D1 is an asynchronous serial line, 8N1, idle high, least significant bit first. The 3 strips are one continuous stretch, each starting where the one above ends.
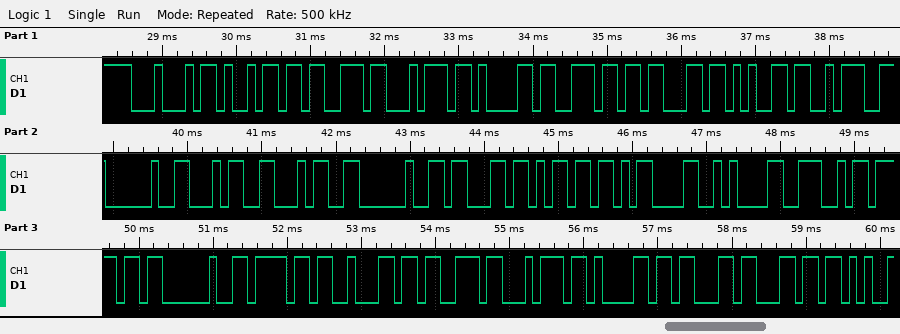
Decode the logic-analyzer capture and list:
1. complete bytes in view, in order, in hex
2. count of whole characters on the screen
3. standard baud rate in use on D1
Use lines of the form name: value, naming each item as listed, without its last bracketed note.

complete bytes in view, in order, in hex: 44 69 73 74 61 6E 63 65 3A 20 34 34 20 63 6D 0D 0A 4E 6F 20 6F 62 73 74 61 63 6C
count of whole characters on the screen: 27
standard baud rate in use on D1: 9600 baud
